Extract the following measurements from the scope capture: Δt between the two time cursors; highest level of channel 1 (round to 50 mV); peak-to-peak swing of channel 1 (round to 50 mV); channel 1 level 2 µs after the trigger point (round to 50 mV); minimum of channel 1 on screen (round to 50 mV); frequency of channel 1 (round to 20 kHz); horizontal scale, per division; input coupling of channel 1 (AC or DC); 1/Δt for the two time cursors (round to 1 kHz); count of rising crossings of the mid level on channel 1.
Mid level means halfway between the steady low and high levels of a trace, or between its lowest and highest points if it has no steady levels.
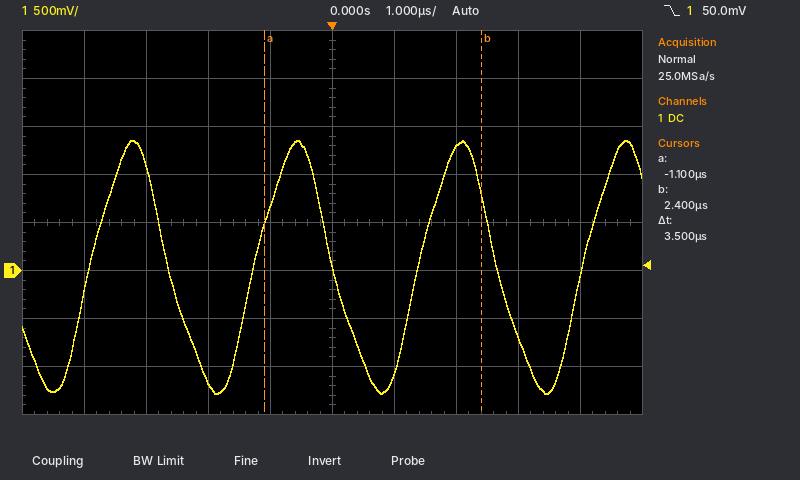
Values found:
3.5 µs
1.35 V
2.65 V
1.30 V
-1.30 V
380 kHz
1 µs
DC
286 kHz
4
